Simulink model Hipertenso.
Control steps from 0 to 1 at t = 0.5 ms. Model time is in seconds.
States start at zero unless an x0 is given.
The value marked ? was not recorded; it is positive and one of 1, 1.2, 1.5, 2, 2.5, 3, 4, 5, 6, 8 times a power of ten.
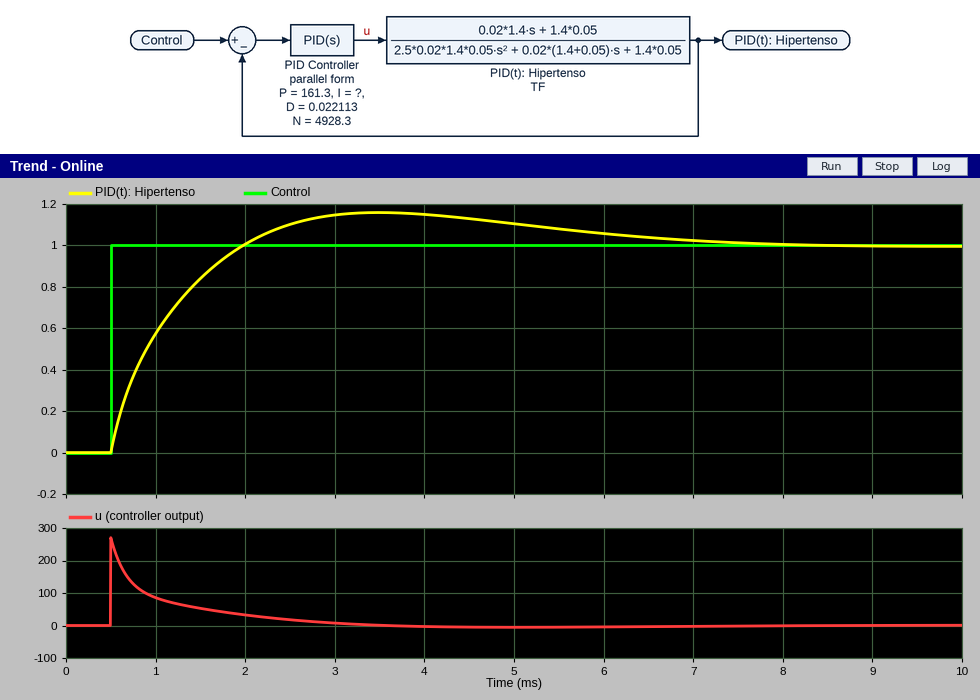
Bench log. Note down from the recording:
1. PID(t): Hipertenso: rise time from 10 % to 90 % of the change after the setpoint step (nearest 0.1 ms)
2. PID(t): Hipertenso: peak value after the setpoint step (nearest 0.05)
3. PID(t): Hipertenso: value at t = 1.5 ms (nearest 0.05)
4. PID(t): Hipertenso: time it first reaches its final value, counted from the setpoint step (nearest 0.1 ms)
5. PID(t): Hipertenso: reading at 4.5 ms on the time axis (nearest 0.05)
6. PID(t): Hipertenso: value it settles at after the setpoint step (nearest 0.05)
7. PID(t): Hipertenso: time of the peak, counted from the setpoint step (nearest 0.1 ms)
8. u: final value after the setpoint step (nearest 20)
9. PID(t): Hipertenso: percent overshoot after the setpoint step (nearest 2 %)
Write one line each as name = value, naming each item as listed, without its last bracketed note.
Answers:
PID(t): Hipertenso: rise time from 10 % to 90 % of the change after the setpoint step = 1.1 ms
PID(t): Hipertenso: peak value after the setpoint step = 1.15
PID(t): Hipertenso: value at t = 1.5 ms = 0.85
PID(t): Hipertenso: time it first reaches its final value, counted from the setpoint step = 1.5 ms
PID(t): Hipertenso: reading at 4.5 ms on the time axis = 1.15
PID(t): Hipertenso: value it settles at after the setpoint step = 1.00
PID(t): Hipertenso: time of the peak, counted from the setpoint step = 3.0 ms
u: final value after the setpoint step = 0
PID(t): Hipertenso: percent overshoot after the setpoint step = 16 %
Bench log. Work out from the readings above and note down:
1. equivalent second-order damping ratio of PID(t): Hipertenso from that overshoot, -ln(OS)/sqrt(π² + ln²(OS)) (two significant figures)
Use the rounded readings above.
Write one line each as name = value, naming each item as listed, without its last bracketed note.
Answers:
equivalent second-order damping ratio of PID(t): Hipertenso from that overshoot, -ln(OS)/sqrt(π² + ln²(OS)) = 0.50
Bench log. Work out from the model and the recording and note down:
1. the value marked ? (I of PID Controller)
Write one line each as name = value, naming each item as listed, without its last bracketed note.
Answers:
the value marked ? = 80000
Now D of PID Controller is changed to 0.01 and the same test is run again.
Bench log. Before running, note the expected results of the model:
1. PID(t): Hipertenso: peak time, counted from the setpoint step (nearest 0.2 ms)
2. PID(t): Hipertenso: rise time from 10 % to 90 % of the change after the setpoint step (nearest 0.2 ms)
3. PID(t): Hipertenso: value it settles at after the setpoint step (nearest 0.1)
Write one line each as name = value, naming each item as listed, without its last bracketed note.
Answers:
PID(t): Hipertenso: peak time, counted from the setpoint step = 2.8 ms
PID(t): Hipertenso: rise time from 10 % to 90 % of the change after the setpoint step = 1.0 ms
PID(t): Hipertenso: value it settles at after the setpoint step = 1.0
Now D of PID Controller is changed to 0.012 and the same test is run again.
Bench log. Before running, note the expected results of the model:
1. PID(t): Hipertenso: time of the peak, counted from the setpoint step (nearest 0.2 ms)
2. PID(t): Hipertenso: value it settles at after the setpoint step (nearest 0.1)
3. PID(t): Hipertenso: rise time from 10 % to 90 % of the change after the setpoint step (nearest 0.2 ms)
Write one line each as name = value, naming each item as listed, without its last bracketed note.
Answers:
PID(t): Hipertenso: time of the peak, counted from the setpoint step = 2.8 ms
PID(t): Hipertenso: value it settles at after the setpoint step = 1.0
PID(t): Hipertenso: rise time from 10 % to 90 % of the change after the setpoint step = 1.0 ms
